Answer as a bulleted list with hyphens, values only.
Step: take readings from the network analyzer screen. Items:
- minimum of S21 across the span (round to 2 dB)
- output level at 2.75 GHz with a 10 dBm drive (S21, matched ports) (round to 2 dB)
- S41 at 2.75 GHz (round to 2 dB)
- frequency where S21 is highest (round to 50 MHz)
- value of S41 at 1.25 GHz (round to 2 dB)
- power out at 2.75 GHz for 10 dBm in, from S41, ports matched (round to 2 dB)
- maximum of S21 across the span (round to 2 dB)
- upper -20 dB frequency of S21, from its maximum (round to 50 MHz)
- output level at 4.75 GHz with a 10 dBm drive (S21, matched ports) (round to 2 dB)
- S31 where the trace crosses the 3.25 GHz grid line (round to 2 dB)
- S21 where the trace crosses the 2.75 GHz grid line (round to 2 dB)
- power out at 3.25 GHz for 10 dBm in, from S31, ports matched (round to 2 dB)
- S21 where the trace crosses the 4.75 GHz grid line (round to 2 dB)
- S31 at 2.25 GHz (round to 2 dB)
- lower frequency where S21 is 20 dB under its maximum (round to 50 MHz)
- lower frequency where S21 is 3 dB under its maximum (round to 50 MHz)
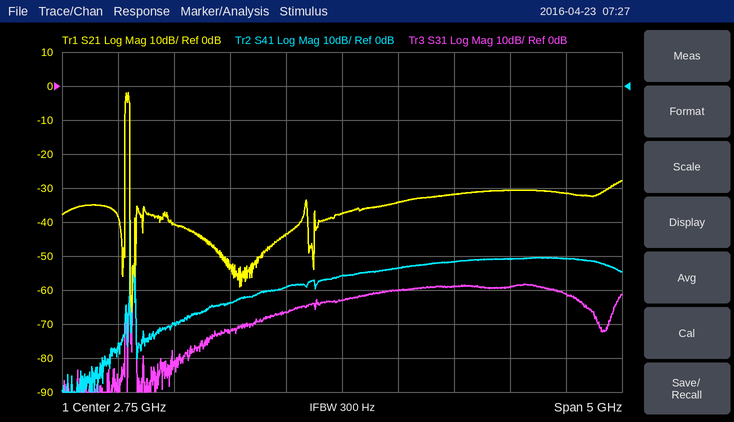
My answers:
- -66 dB
- -28 dBm
- -56 dB
- 850 MHz
- -70 dB
- -46 dBm
- -2 dB
- 850 MHz
- -22 dBm
- -60 dB
- -38 dB
- -50 dBm
- -32 dB
- -66 dB
- 800 MHz
- 850 MHz
